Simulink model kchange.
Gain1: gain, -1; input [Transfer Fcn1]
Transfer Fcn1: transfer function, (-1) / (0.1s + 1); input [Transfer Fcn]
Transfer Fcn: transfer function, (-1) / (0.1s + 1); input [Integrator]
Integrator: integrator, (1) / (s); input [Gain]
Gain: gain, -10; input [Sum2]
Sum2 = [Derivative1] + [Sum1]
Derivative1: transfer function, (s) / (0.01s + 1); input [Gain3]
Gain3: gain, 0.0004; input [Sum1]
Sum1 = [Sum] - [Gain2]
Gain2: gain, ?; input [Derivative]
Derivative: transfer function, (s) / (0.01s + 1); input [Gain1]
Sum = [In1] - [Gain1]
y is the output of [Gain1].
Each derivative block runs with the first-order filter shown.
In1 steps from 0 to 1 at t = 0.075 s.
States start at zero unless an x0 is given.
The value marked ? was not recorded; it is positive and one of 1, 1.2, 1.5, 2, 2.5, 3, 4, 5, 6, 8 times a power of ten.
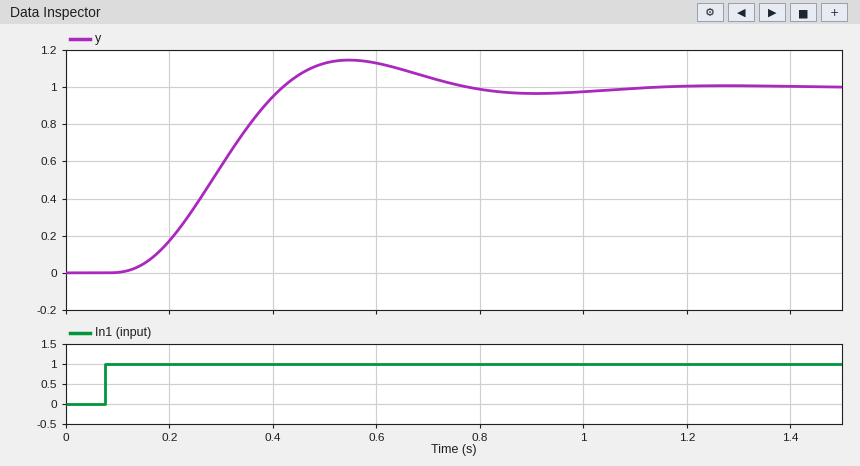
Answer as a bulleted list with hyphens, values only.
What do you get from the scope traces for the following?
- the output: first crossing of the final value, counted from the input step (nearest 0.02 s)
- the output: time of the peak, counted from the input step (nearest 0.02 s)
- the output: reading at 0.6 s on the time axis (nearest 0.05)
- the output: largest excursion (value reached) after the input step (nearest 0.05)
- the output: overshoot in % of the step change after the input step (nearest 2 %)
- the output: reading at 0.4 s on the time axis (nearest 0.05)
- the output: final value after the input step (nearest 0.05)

- 0.34 s
- 0.48 s
- 1.15
- 1.15
- 14 %
- 0.95
- 1.00
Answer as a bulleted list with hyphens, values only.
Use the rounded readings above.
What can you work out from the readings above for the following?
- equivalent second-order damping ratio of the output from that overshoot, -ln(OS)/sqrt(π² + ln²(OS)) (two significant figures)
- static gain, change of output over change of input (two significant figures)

- 0.53
- 1.0
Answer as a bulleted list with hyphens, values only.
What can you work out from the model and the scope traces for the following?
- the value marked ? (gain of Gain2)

- 0.08
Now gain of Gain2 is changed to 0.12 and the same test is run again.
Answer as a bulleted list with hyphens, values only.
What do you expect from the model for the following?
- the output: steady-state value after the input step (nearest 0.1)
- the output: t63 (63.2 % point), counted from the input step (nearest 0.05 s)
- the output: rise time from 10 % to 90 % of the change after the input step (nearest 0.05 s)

- 1.0
- 0.25 s
- 0.25 s
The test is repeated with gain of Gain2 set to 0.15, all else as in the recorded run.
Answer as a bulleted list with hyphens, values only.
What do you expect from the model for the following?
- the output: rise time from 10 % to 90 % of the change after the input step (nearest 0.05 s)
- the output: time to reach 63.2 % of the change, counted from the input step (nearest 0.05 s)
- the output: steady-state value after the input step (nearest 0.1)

- 0.30 s
- 0.25 s
- 1.0
